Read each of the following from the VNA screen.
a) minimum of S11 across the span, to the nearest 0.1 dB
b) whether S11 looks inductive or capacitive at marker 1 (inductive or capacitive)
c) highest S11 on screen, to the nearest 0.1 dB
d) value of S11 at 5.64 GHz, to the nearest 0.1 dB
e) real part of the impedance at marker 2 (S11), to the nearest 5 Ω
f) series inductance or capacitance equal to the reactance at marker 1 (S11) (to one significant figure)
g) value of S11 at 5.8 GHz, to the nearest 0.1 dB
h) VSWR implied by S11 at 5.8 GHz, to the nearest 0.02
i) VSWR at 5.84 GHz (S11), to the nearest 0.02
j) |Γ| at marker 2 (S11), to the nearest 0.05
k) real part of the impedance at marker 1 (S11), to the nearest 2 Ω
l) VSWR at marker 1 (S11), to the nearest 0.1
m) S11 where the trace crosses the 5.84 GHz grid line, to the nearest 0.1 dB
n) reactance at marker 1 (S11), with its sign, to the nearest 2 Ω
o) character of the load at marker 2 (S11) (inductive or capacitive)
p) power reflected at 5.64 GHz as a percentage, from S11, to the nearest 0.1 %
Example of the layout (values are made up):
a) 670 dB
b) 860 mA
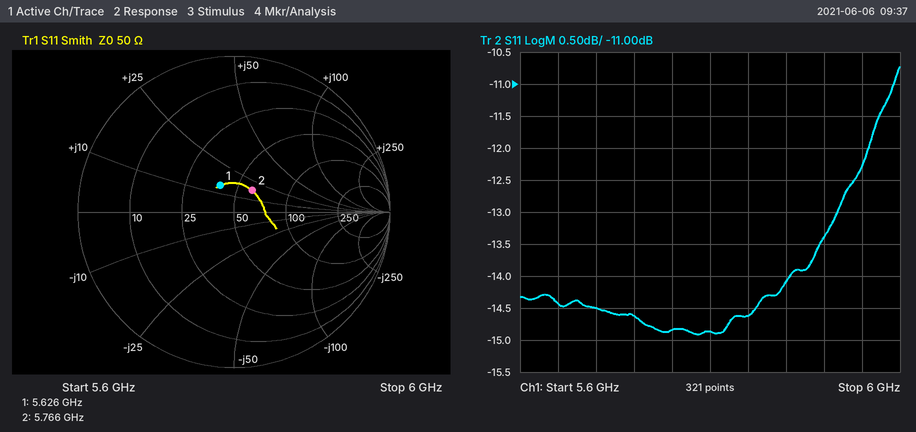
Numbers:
a) -14.9 dB
b) inductive
c) -10.7 dB
d) -14.4 dB
e) 60 Ω
f) 400 pH
g) -14.9 dB
h) 1.44
i) 1.46
j) 0.20
k) 40 Ω
l) 1.5
m) -14.6 dB
n) +14 Ω
o) inductive
p) 3.6 %
